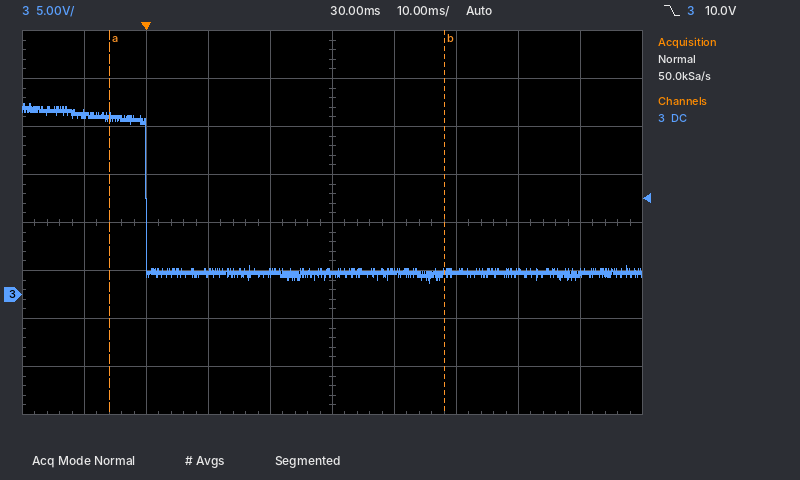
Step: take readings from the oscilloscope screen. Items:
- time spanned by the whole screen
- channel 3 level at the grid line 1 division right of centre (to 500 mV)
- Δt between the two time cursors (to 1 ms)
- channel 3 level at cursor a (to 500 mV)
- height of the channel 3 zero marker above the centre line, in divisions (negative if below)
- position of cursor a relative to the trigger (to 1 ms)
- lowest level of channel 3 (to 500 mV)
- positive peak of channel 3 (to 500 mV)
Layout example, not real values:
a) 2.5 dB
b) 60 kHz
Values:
a) 100 ms
b) 2.5 V
c) 54 ms
d) 18.5 V
e) -1.5 div
f) -6 ms
g) 1.0 V
h) 20.0 V
